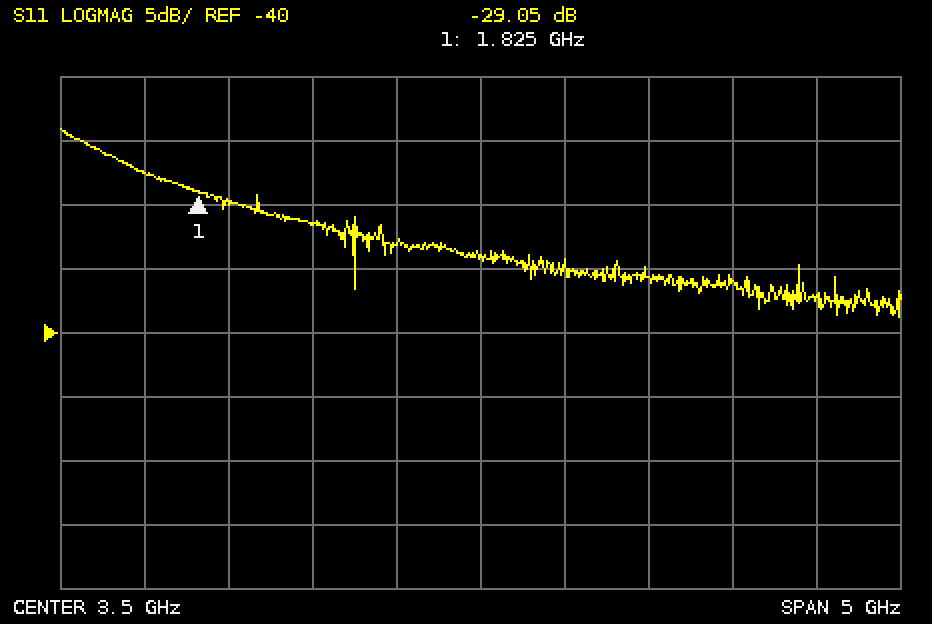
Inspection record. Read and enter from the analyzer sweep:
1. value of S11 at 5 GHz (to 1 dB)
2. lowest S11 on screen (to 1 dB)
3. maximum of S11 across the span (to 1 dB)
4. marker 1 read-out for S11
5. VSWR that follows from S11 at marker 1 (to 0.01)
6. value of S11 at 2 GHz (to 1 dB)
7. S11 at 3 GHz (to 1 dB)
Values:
-36 dB
-39 dB
-24 dB
-29.05 dB
1.07
-30 dB
-33 dB
